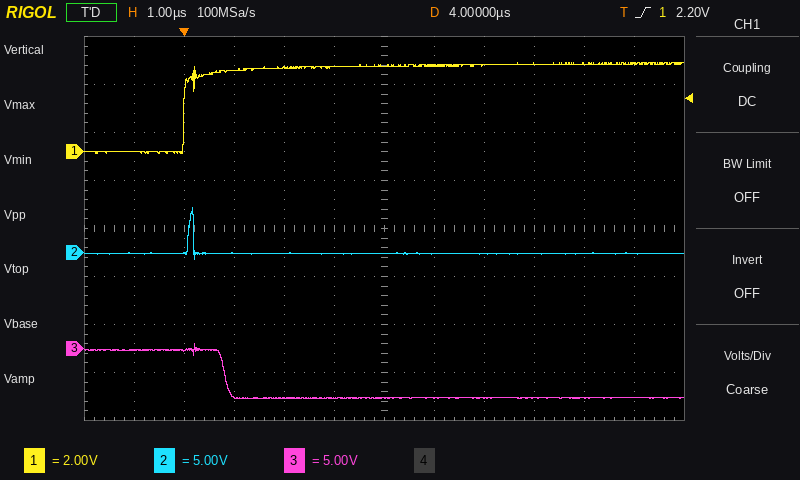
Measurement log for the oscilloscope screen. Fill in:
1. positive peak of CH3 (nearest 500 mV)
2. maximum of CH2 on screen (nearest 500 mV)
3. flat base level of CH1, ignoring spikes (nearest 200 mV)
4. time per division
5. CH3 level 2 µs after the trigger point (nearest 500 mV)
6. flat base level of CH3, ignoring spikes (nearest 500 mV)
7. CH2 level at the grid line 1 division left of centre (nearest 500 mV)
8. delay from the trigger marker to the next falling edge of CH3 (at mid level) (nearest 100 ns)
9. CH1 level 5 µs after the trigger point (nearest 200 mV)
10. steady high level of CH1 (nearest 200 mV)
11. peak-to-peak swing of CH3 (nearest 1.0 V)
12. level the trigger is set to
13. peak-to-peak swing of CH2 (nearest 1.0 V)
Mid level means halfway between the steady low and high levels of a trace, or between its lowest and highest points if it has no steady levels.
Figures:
500 mV
4.5 V
0.0 V
1 µs
-5.0 V
-5.0 V
0.0 V
800 ns
3.6 V
3.6 V
6.0 V
2.20 V
5.0 V
